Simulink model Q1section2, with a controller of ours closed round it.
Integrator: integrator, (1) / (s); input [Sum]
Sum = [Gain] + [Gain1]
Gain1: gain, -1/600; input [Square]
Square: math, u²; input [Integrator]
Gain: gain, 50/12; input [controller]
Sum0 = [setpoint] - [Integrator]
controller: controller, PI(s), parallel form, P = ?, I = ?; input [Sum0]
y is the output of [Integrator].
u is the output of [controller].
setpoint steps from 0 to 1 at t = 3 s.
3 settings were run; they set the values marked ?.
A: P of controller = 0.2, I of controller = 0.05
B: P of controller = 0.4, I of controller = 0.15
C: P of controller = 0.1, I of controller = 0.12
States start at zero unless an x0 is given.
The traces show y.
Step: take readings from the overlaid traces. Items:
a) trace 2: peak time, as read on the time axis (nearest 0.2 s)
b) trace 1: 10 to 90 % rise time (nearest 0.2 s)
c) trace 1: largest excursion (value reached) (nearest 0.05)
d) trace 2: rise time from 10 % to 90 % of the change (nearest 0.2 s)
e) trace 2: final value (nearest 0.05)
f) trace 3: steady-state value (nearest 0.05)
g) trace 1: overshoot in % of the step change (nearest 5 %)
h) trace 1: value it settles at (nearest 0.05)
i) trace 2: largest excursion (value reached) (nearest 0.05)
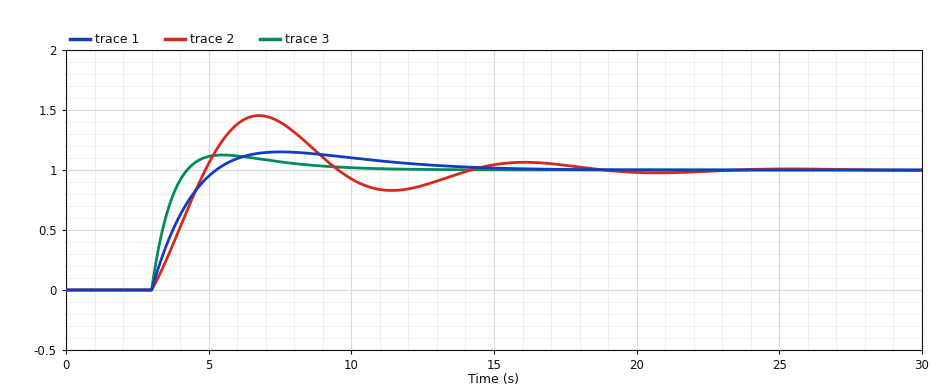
6.8 s
1.6 s
1.15
1.4 s
1.00
1.00
15 %
1.00
1.45
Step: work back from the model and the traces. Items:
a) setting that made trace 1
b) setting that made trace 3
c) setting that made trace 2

A
B
C
